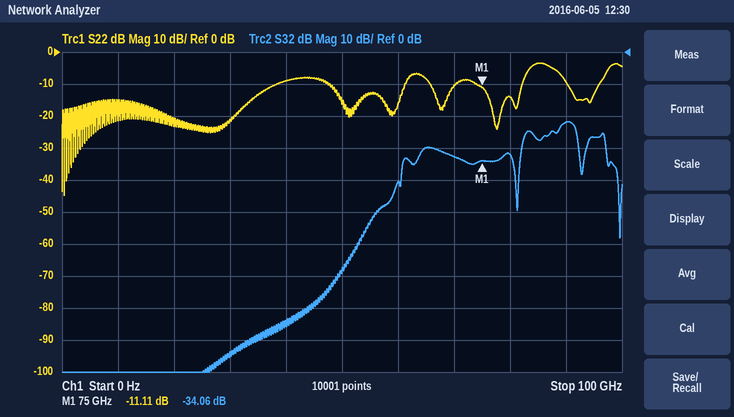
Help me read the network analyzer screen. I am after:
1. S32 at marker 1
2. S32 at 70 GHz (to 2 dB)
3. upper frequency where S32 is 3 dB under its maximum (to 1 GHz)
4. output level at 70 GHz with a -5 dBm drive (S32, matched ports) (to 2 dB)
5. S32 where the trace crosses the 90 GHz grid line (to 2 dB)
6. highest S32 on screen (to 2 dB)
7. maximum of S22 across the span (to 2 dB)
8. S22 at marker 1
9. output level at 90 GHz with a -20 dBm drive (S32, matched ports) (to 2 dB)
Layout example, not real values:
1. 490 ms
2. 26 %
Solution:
1. -34.06 dB
2. -32 dB
3. 92 GHz
4. -38 dBm
5. -22 dB
6. -22 dB
7. -4 dB
8. -11.11 dB
9. -42 dBm
